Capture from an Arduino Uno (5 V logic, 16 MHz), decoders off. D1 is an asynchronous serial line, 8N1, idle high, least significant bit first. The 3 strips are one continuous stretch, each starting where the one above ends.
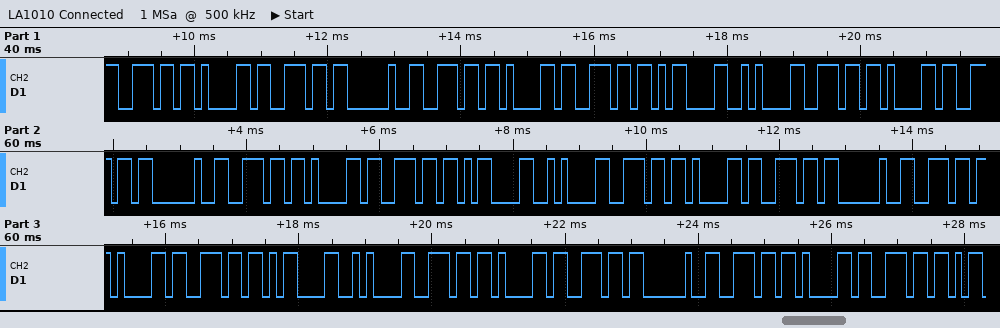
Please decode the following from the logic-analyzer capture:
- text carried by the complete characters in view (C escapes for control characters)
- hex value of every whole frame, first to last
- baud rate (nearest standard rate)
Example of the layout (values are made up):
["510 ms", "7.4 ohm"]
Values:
["\"nan nan\\r\\nnan nan\\r\\nnan nan\\r\\nnan nan\"", "6E 61 6E 20 6E 61 6E 0D 0A 6E 61 6E 20 6E 61 6E 0D 0A 6E 61 6E 20 6E 61 6E 0D 0A 6E 61 6E 20 6E 61 6E", "9600 baud"]
